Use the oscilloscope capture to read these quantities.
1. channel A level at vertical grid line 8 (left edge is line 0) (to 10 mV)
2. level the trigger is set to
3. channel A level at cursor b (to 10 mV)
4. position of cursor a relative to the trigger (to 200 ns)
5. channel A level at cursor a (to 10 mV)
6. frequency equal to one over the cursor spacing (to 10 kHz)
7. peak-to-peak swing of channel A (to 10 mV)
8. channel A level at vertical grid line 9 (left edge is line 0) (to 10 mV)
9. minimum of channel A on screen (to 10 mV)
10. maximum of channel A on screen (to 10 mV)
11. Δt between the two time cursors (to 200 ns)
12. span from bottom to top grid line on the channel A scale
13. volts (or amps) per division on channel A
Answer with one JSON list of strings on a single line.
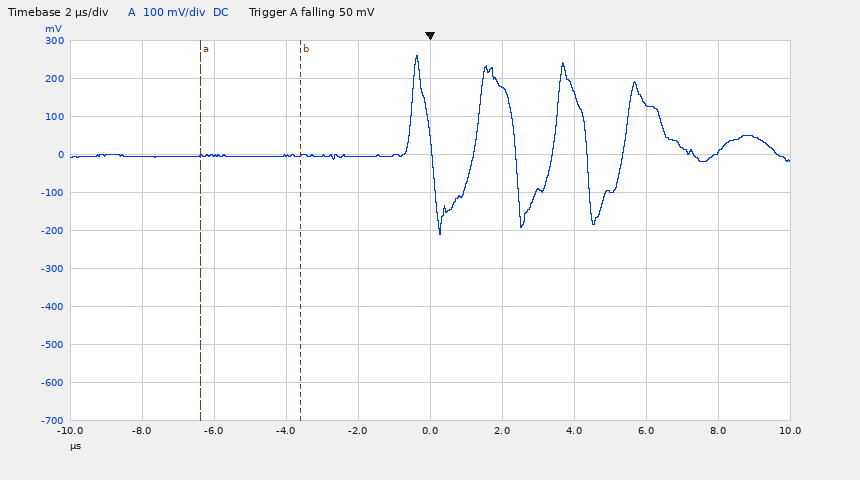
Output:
["130 mV", "50 mV", "0 mV", "-6.4 µs", "0 mV", "360 kHz", "470 mV", "10 mV", "-210 mV", "260 mV", "2.8 µs", "1 V", "100 mV"]
